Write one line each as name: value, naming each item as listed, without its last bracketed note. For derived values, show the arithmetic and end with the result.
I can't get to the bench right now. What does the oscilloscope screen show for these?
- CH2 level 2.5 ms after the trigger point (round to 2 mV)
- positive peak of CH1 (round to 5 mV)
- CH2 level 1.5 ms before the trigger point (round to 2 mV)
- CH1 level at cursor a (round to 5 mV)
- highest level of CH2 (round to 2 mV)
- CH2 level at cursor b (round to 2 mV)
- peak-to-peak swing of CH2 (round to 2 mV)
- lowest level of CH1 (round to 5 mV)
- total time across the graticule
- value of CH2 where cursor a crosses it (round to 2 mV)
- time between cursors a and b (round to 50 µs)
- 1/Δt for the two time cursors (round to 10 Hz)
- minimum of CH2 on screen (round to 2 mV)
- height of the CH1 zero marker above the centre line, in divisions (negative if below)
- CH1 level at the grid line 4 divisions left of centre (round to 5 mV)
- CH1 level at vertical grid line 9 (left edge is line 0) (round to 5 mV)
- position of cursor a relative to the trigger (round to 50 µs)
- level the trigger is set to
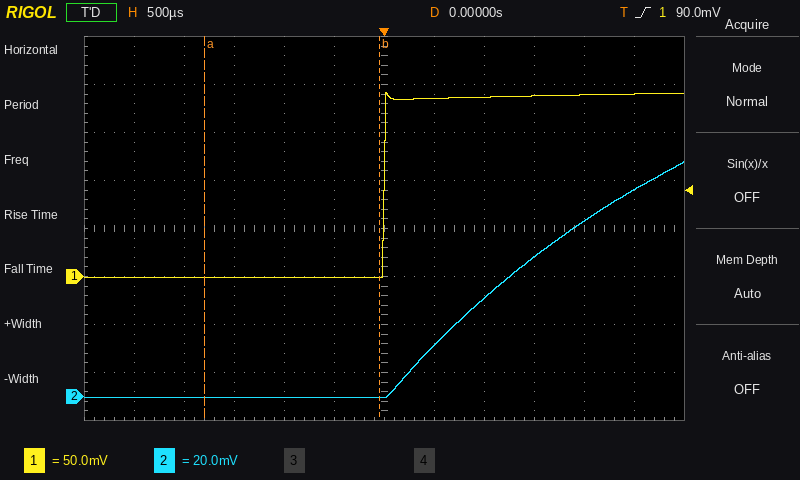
CH2 level 2.5 ms after the trigger point: 86 mV
positive peak of CH1: 190 mV
CH2 level 1.5 ms before the trigger point: 0 mV
CH1 level at cursor a: 0 mV
highest level of CH2: 98 mV
CH2 level at cursor b: 0 mV
peak-to-peak swing of CH2: 98 mV − (0 mV) = 98 mV
lowest level of CH1: 0 mV
total time across the graticule: 6 ms
value of CH2 where cursor a crosses it: 0 mV
time between cursors a and b: 1.75 ms
1/Δt for the two time cursors: 1 / 1.75 ms ≈ 570 Hz
minimum of CH2 on screen: 0 mV
height of the CH1 zero marker above the centre line, in divisions: -1.0 div
CH1 level at the grid line 4 divisions left of centre: 0 mV
CH1 level at vertical grid line 9 (left edge is line 0): 190 mV
position of cursor a relative to the trigger: -1.80 ms
level the trigger is set to: 90.0 mV
